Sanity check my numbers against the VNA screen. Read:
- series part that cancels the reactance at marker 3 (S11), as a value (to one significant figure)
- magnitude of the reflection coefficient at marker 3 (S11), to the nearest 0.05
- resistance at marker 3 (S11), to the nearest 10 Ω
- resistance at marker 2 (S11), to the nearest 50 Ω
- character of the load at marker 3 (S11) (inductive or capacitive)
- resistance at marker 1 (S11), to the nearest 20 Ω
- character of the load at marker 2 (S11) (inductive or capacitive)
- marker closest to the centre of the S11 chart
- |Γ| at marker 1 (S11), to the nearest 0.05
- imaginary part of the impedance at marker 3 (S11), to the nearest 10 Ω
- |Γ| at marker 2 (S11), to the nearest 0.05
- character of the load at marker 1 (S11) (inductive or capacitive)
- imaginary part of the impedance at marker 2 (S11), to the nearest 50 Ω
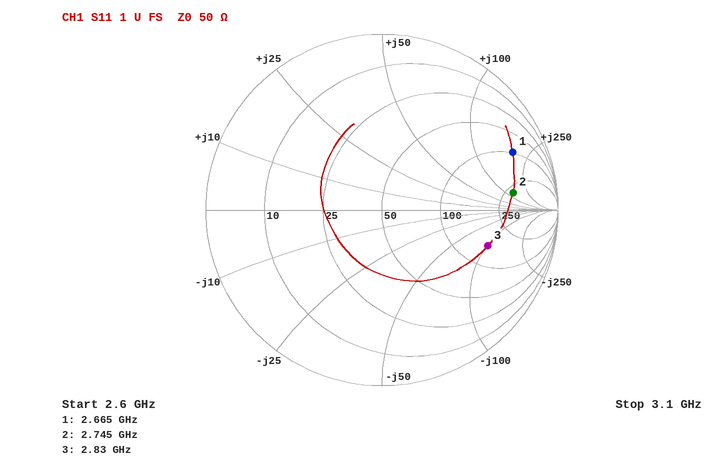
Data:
6 nH
0.65
150 Ω
300 Ω
capacitive
100 Ω
inductive
marker 3
0.80
-100 Ω
0.75
inductive
+150 Ω
